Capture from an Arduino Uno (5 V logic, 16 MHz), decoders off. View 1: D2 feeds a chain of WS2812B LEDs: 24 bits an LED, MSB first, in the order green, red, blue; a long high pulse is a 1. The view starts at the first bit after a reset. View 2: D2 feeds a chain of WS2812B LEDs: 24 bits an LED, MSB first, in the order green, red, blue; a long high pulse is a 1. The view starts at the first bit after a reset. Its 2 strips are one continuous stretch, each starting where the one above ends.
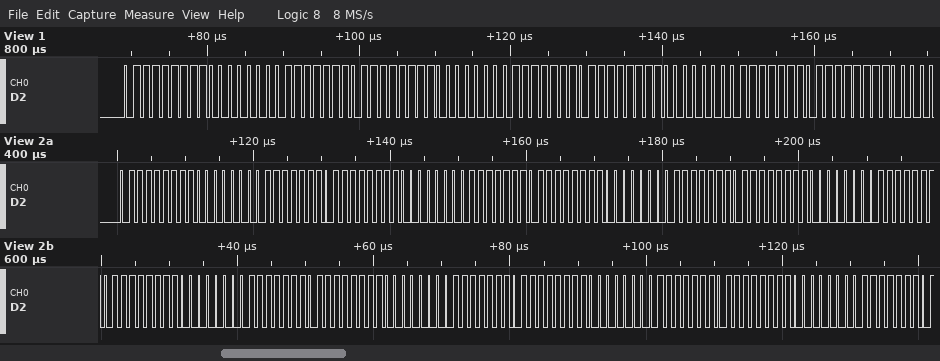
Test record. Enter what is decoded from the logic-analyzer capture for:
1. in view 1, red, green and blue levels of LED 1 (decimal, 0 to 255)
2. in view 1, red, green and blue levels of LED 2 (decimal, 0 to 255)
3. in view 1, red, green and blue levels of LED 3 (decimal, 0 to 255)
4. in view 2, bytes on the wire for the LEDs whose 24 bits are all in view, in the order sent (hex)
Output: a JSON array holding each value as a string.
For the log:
["128, 127, 127", "128, 127, 127", "128, 127, 127", "7F 80 7F 7F 80 7F 7F 80 7F 7F 80 7F 7F 80 7F 7F 80 7F 7F 80 7F 7F 80 7F"]
